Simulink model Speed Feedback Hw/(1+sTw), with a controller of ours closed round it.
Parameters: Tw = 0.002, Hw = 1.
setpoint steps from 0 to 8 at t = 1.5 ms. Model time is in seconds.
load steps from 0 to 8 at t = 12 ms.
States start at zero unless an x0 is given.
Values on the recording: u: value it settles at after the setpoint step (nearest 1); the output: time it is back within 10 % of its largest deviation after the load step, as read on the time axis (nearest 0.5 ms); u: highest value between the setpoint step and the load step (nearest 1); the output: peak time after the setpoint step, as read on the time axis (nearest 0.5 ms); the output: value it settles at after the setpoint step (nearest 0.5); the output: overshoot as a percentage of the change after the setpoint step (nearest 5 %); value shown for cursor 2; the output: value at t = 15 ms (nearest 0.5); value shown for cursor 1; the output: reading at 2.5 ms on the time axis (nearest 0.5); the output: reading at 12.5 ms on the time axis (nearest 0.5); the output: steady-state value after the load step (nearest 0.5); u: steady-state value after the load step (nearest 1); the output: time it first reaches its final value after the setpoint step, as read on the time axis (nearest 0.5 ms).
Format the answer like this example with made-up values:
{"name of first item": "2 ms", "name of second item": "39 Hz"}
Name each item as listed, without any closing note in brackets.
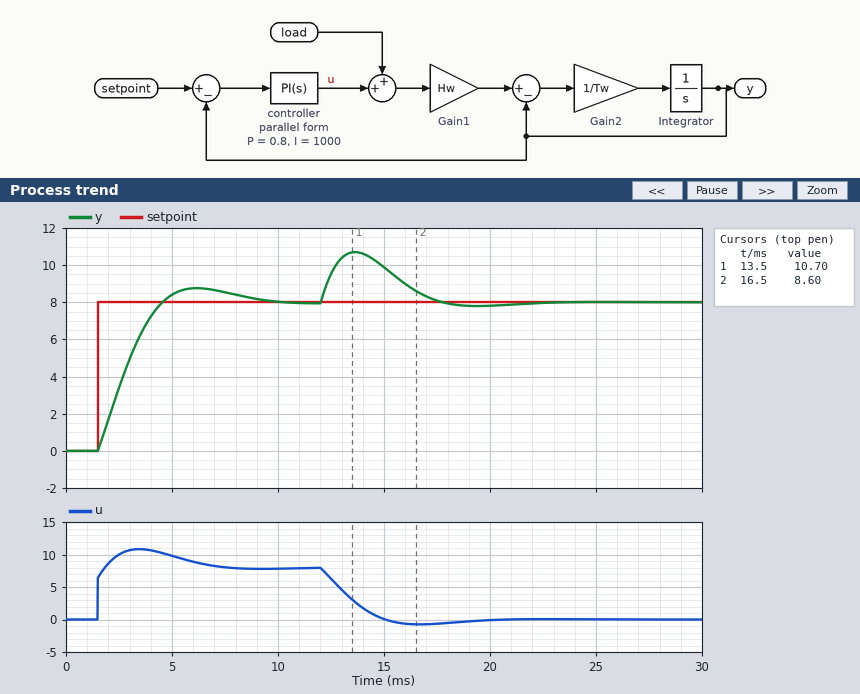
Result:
{"u: value it settles at after the setpoint step": "8", "the output: time it is back within 10 % of its largest deviation after the load step, as read on the time axis": "17.0 ms", "u: highest value between the setpoint step and the load step": "11", "the output: peak time after the setpoint step, as read on the time axis": "6.0 ms", "the output: value it settles at after the setpoint step": "8.0", "the output: overshoot as a percentage of the change after the setpoint step": "10 %", "value shown for cursor 2": "8.60", "the output: value at t = 15 ms": "10.0", "value shown for cursor 1": "10.70", "the output: reading at 2.5 ms on the time axis": "3.5", "the output: reading at 12.5 ms on the time axis": "9.5", "the output: steady-state value after the load step": "8.0", "u: steady-state value after the load step": "0", "the output: time it first reaches its final value after the setpoint step, as read on the time axis": "4.5 ms"}
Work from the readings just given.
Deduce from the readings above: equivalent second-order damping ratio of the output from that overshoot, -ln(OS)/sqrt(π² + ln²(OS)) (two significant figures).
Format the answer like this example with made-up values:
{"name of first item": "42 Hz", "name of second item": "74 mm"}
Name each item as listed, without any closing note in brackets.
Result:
{"equivalent second-order damping ratio of the output from that overshoot, -ln(OS)/sqrt(π² + ln²(OS))": "0.59"}
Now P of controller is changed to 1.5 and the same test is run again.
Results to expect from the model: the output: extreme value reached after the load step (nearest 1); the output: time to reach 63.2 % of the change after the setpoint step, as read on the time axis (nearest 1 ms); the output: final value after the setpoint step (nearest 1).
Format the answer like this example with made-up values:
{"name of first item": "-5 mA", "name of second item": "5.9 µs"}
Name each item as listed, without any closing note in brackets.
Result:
{"the output: extreme value reached after the load step": "10", "the output: time to reach 63.2 % of the change after the setpoint step, as read on the time axis": "3 ms", "the output: final value after the setpoint step": "8"}
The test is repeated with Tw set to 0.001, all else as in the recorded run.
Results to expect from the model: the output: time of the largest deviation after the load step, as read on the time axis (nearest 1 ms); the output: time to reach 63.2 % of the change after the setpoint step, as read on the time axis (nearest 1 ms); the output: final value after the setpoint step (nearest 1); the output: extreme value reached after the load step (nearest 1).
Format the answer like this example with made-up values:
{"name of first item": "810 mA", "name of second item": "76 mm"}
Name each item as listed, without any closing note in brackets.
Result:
{"the output: time of the largest deviation after the load step, as read on the time axis": "13 ms", "the output: time to reach 63.2 % of the change after the setpoint step, as read on the time axis": "3 ms", "the output: final value after the setpoint step": "8", "the output: extreme value reached after the load step": "11"}
